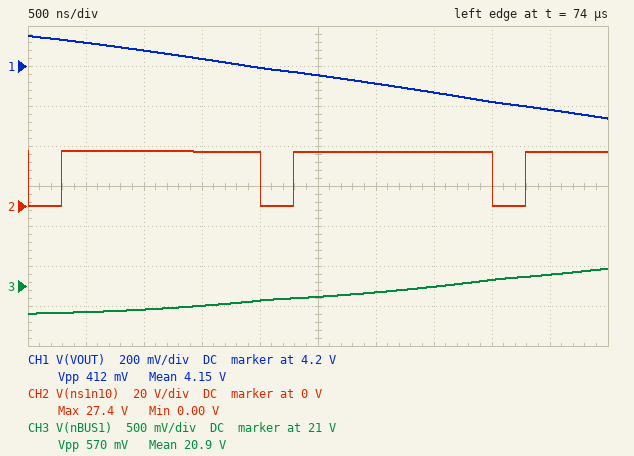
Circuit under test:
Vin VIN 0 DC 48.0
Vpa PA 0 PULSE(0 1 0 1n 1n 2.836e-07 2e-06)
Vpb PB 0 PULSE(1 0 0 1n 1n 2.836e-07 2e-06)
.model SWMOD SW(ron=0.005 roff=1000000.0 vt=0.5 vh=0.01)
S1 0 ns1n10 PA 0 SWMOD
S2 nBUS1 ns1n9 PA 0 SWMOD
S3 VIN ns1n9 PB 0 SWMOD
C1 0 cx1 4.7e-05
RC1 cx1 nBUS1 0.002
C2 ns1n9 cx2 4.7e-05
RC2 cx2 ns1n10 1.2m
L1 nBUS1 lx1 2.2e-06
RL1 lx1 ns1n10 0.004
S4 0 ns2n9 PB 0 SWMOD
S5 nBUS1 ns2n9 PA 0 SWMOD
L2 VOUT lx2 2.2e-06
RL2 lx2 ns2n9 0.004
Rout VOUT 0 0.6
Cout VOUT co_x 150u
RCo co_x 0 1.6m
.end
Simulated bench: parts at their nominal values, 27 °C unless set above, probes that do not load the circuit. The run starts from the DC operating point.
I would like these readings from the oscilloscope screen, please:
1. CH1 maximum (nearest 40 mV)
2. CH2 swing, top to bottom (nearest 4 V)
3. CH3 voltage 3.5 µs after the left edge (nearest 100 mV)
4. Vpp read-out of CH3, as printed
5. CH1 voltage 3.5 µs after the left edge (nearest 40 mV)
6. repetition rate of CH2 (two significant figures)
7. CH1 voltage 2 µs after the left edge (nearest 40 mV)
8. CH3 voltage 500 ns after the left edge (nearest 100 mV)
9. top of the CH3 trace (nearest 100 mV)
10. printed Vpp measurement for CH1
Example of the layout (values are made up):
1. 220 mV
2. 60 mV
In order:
1. 4.36 V
2. 28 V
3. 21.0 V
4. 570 mV
5. 4.08 V
6. 500 kHz
7. 4.20 V
8. 20.7 V
9. 21.2 V
10. 412 mV
